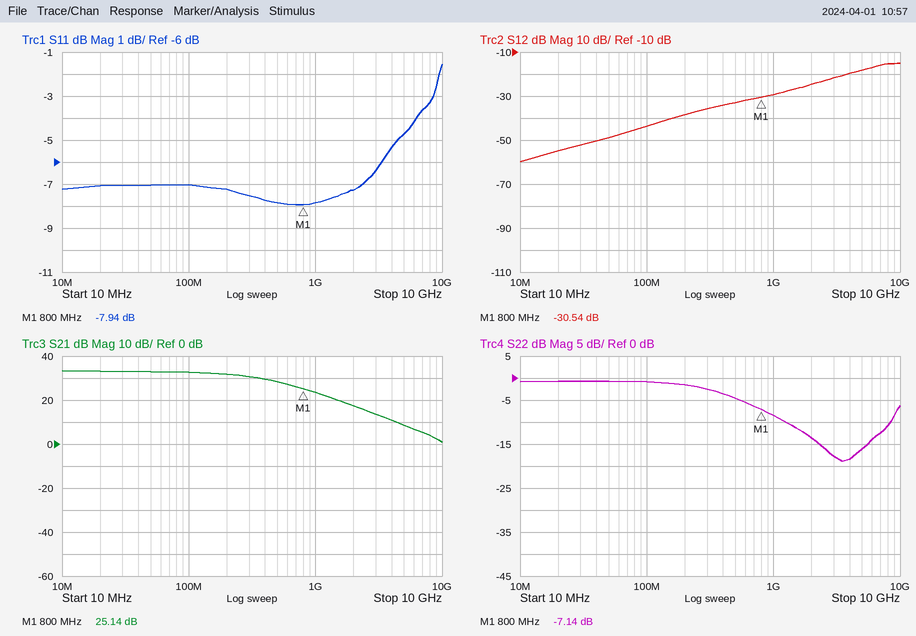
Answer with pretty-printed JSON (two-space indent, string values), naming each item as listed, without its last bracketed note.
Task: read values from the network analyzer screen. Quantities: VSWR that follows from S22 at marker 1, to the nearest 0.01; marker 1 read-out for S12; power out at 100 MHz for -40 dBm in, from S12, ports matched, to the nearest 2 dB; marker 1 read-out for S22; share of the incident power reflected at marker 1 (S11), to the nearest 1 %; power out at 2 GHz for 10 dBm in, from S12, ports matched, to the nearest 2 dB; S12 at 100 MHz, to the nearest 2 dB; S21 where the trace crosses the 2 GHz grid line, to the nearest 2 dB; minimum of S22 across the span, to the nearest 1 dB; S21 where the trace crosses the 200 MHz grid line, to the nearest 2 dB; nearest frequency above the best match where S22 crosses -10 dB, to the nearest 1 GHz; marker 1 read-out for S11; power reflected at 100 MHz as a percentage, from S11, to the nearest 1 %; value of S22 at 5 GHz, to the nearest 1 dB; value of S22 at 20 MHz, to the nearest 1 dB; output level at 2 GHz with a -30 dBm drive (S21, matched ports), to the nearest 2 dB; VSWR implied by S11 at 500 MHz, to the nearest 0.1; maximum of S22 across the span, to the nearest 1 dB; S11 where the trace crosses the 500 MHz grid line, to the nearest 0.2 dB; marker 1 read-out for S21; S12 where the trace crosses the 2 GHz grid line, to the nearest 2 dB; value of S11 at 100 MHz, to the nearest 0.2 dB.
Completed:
{
  "VSWR that follows from S22 at marker 1, to the nearest 0.01": "2.57",
  "marker 1 read-out for S12": "-30.54 dB",
  "power out at 100 MHz for -40 dBm in, from S12, ports matched, to the nearest 2 dB": "-84 dBm",
  "marker 1 read-out for S22": "-7.14 dB",
  "share of the incident power reflected at marker 1 (S11), to the nearest 1 %": "16 %",
  "power out at 2 GHz for 10 dBm in, from S12, ports matched, to the nearest 2 dB": "-14 dBm",
  "S12 at 100 MHz, to the nearest 2 dB": "-44 dB",
  "S21 where the trace crosses the 2 GHz grid line, to the nearest 2 dB": "18 dB",
  "minimum of S22 across the span, to the nearest 1 dB": "-19 dB",
  "S21 where the trace crosses the 200 MHz grid line, to the nearest 2 dB": "32 dB",
  "nearest frequency above the best match where S22 crosses -10 dB, to the nearest 1 GHz": "8 GHz",
  "marker 1 read-out for S11": "-7.94 dB",
  "power reflected at 100 MHz as a percentage, from S11, to the nearest 1 %": "20 %",
  "value of S22 at 5 GHz, to the nearest 1 dB": "-16 dB",
  "value of S22 at 20 MHz, to the nearest 1 dB": "-1 dB",
  "output level at 2 GHz with a -30 dBm drive (S21, matched ports), to the nearest 2 dB": "-12 dBm",
  "VSWR implied by S11 at 500 MHz, to the nearest 0.1": "2.4",
  "maximum of S22 across the span, to the nearest 1 dB": "-1 dB",
  "S11 where the trace crosses the 500 MHz grid line, to the nearest 0.2 dB": "-7.8 dB",
  "marker 1 read-out for S21": "25.14 dB",
  "S12 where the trace crosses the 2 GHz grid line, to the nearest 2 dB": "-24 dB",
  "value of S11 at 100 MHz, to the nearest 0.2 dB": "-7.0 dB"
}
